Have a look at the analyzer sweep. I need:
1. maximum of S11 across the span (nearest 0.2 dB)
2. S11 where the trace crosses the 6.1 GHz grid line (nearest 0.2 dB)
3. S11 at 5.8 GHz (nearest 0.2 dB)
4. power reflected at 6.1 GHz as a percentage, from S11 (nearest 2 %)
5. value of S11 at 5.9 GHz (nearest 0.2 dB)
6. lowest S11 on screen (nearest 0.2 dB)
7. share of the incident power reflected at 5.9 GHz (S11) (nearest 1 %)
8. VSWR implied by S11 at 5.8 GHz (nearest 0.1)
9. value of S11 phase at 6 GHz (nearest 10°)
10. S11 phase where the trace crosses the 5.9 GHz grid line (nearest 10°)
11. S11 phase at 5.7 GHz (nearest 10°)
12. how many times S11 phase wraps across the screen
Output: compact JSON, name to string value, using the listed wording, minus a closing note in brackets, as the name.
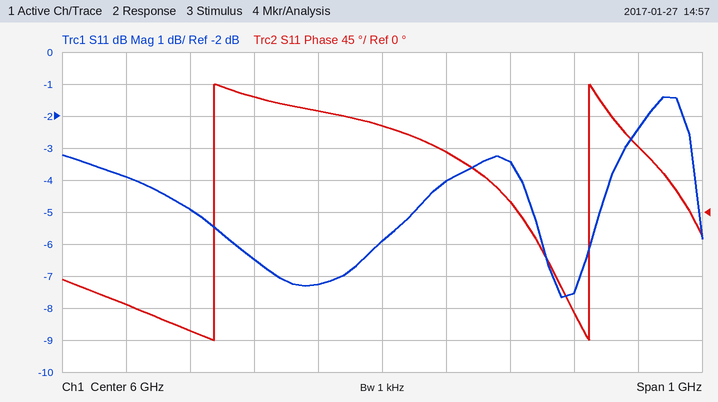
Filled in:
{"maximum of S11 across the span": "-1.4 dB", "S11 where the trace crosses the 6.1 GHz grid line": "-4.0 dB", "S11 at 5.8 GHz": "-6.4 dB", "power reflected at 6.1 GHz as a percentage, from S11": "40 %", "value of S11 at 5.9 GHz": "-7.2 dB", "lowest S11 on screen": "-7.6 dB", "share of the incident power reflected at 5.9 GHz (S11)": "19 %", "VSWR implied by S11 at 5.8 GHz": "2.8", "value of S11 phase at 6 GHz": "120°", "S11 phase where the trace crosses the 5.9 GHz grid line": "140°", "S11 phase at 5.7 GHz": "-170°", "how many times S11 phase wraps across the screen": "2"}
